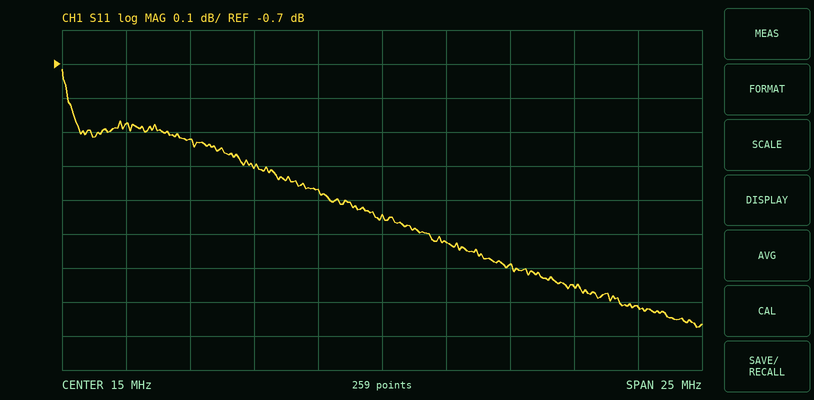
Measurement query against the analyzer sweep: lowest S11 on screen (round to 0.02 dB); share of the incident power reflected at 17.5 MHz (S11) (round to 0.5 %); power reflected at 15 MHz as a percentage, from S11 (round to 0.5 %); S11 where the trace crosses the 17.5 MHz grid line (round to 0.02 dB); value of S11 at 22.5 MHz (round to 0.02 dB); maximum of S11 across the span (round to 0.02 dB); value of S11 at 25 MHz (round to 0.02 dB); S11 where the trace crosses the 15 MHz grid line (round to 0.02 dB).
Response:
-1.48 dB
75.5 %
77.0 %
-1.22 dB
-1.36 dB
-0.72 dB
-1.42 dB
-1.14 dB
